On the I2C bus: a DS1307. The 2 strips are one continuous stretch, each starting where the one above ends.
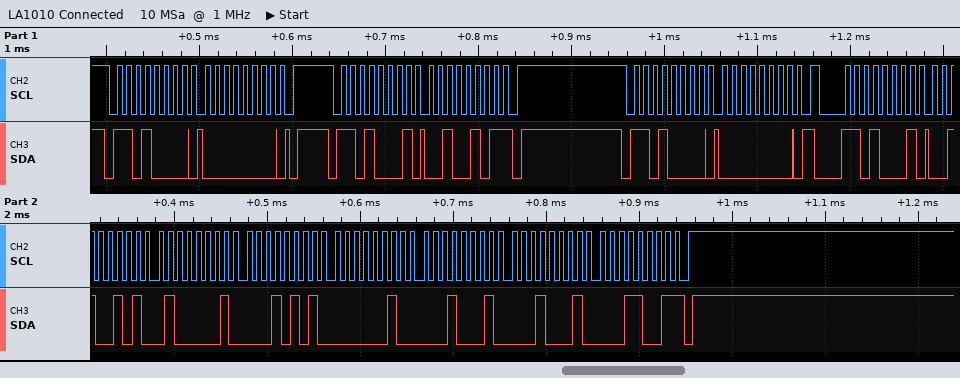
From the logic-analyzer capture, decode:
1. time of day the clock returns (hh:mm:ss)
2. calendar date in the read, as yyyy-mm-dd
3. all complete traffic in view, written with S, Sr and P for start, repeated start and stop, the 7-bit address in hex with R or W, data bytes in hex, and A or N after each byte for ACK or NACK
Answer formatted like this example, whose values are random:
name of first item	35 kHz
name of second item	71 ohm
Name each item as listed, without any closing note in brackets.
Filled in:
time of day the clock returns	15:41:25
calendar date in the read, as yyyy-mm-dd	2019-11-11
all complete traffic in view, written with S, Sr and P for start, repeated start and stop, the 7-bit address in hex with R or W, data bytes in hex, and A or N after each byte for ACK or NACK	S 68W A 00 A P S 68R A 25 N P S 68W A 00 A Sr 68R A 25 A 41 A 15 A 02 A 11 A 11 A 19 N P
